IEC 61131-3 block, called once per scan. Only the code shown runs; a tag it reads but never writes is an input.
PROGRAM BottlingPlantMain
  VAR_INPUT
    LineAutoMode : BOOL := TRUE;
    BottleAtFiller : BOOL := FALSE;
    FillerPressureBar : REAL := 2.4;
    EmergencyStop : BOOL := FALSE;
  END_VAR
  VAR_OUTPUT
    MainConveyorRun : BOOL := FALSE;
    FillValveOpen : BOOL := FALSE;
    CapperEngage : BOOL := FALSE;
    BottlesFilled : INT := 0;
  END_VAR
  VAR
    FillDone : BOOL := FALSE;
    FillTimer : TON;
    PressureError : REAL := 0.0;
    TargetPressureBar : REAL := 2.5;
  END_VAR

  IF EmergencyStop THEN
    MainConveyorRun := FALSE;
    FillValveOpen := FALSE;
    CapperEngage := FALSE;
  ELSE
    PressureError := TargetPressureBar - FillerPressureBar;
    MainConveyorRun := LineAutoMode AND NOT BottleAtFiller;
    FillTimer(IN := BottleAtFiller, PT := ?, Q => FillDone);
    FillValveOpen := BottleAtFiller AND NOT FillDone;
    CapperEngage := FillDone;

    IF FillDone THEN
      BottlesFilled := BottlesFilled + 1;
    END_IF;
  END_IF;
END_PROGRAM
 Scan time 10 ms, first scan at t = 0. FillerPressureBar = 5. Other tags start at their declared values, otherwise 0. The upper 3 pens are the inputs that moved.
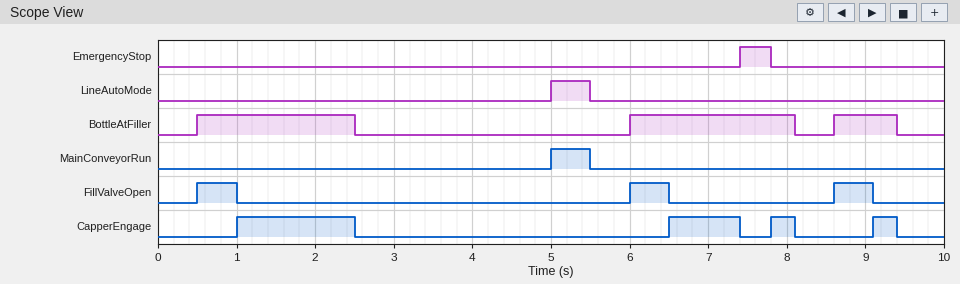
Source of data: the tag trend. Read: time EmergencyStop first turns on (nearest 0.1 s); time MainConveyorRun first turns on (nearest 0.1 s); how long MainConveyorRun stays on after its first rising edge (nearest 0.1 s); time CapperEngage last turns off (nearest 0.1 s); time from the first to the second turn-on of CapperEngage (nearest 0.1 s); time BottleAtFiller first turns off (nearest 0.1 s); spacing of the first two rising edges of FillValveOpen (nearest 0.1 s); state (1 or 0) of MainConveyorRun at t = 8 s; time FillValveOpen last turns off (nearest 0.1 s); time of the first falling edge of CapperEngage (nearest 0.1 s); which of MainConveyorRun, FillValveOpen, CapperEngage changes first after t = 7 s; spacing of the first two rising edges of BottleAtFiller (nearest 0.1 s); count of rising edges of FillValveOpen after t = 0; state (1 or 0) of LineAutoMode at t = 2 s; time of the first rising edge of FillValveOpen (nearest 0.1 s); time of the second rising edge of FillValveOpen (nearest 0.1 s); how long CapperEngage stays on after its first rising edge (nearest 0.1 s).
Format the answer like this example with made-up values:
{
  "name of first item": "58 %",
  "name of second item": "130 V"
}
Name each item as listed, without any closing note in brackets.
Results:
{
  "time EmergencyStop first turns on": "7.4 s",
  "time MainConveyorRun first turns on": "5.0 s",
  "how long MainConveyorRun stays on after its first rising edge": "0.5 s",
  "time CapperEngage last turns off": "9.4 s",
  "time from the first to the second turn-on of CapperEngage": "5.5 s",
  "time BottleAtFiller first turns off": "2.5 s",
  "spacing of the first two rising edges of FillValveOpen": "5.5 s",
  "state (1 or 0) of MainConveyorRun at t = 8 s": "0",
  "time FillValveOpen last turns off": "9.1 s",
  "time of the first falling edge of CapperEngage": "2.5 s",
  "which of MainConveyorRun, FillValveOpen, CapperEngage changes first after t = 7 s": "CapperEngage",
  "spacing of the first two rising edges of BottleAtFiller": "5.5 s",
  "count of rising edges of FillValveOpen after t = 0": "3",
  "state (1 or 0) of LineAutoMode at t = 2 s": "0",
  "time of the first rising edge of FillValveOpen": "0.5 s",
  "time of the second rising edge of FillValveOpen": "6.0 s",
  "how long CapperEngage stays on after its first rising edge": "1.5 s"
}
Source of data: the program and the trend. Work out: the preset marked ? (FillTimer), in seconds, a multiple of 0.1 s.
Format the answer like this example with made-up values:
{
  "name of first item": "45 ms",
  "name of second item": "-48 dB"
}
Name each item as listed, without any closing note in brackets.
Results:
{
  "the preset marked ? (FillTimer), in seconds, a multiple of 0.1 s": "0.5 s"
}
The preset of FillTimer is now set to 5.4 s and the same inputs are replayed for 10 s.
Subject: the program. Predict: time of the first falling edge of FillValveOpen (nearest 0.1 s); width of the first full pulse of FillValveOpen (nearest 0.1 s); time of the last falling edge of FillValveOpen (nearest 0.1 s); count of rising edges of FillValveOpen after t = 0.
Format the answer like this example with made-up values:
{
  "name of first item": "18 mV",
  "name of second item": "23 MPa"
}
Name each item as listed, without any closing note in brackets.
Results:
{
  "time of the first falling edge of FillValveOpen": "2.5 s",
  "width of the first full pulse of FillValveOpen": "2.0 s",
  "time of the last falling edge of FillValveOpen": "9.4 s",
  "count of rising edges of FillValveOpen after t = 0": "4"
}
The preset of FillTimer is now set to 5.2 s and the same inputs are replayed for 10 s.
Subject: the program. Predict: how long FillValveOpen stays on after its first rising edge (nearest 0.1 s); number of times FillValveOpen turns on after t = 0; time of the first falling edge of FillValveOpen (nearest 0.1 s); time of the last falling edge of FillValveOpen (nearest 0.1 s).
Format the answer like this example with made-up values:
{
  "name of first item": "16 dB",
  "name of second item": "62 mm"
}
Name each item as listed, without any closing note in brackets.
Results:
{
  "how long FillValveOpen stays on after its first rising edge": "2.0 s",
  "number of times FillValveOpen turns on after t = 0": "4",
  "time of the first falling edge of FillValveOpen": "2.5 s",
  "time of the last falling edge of FillValveOpen": "9.4 s"
}
